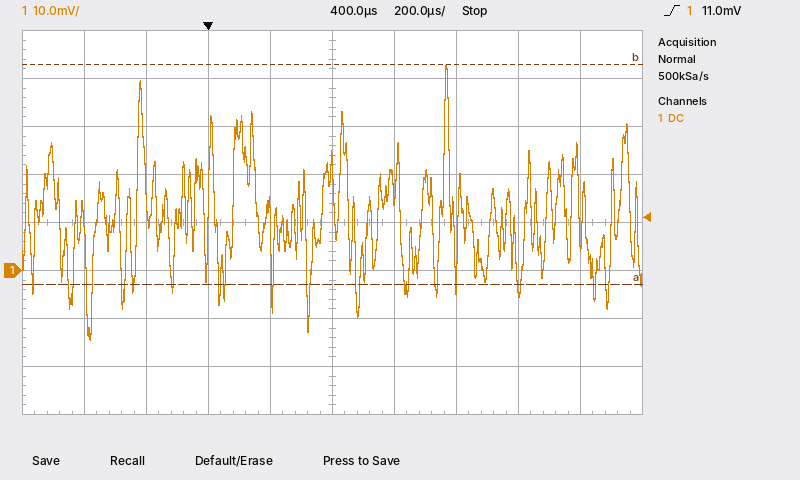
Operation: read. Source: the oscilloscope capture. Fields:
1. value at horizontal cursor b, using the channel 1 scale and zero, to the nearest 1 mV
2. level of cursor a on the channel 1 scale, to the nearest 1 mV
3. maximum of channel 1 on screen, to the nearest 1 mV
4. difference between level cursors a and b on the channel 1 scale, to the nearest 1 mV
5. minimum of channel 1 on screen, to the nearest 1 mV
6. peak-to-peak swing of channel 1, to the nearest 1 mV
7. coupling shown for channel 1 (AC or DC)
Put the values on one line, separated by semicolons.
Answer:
43 mV; -3 mV; 43 mV; 46 mV; -14 mV; 57 mV; DC
